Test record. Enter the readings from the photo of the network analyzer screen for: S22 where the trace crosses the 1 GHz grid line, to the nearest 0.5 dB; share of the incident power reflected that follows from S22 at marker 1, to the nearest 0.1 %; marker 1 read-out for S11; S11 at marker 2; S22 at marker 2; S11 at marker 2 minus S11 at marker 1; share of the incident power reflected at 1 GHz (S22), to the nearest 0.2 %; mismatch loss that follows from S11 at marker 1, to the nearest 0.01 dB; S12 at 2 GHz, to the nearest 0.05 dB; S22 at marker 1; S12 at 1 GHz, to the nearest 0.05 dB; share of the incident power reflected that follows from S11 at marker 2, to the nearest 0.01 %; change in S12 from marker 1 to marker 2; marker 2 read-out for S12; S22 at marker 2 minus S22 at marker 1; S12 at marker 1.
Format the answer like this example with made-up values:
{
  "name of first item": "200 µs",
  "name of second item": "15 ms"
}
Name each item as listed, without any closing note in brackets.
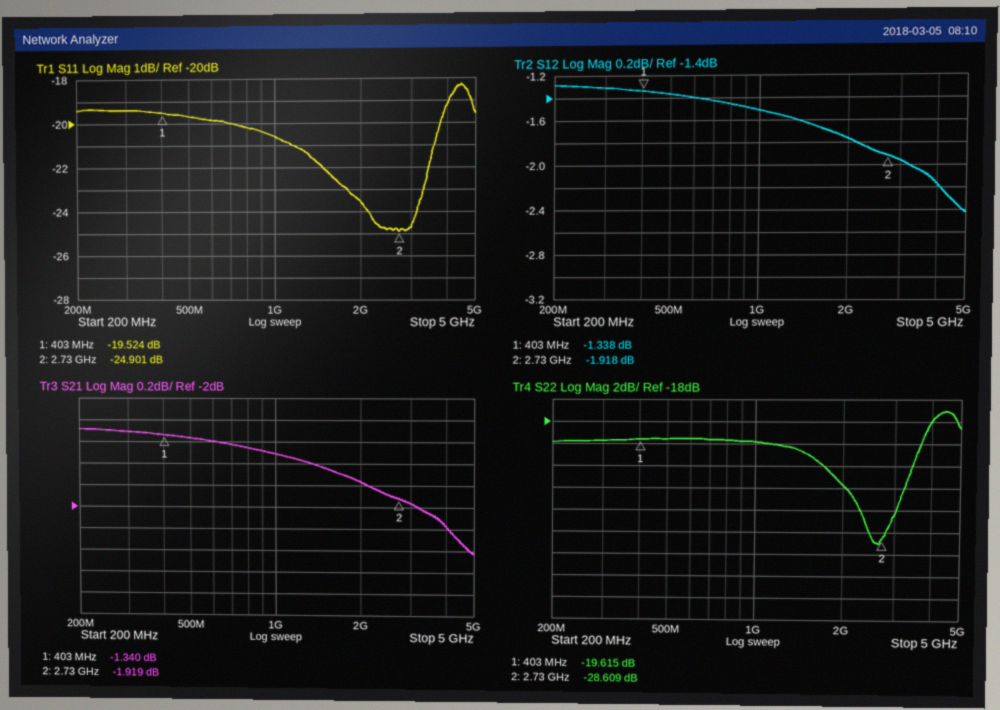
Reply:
{
  "S22 where the trace crosses the 1 GHz grid line, to the nearest 0.5 dB": "-20.0 dB",
  "share of the incident power reflected that follows from S22 at marker 1, to the nearest 0.1 %": "1.1 %",
  "marker 1 read-out for S11": "-19.524 dB",
  "S11 at marker 2": "-24.901 dB",
  "S22 at marker 2": "-28.609 dB",
  "S11 at marker 2 minus S11 at marker 1": "-5.377 dB",
  "share of the incident power reflected at 1 GHz (S22), to the nearest 0.2 %": "1.0 %",
  "mismatch loss that follows from S11 at marker 1, to the nearest 0.01 dB": "0.05 dB",
  "S12 at 2 GHz, to the nearest 0.05 dB": "-1.75 dB",
  "S22 at marker 1": "-19.615 dB",
  "S12 at 1 GHz, to the nearest 0.05 dB": "-1.50 dB",
  "share of the incident power reflected that follows from S11 at marker 2, to the nearest 0.01 %": "0.32 %",
  "change in S12 from marker 1 to marker 2": "-0.580 dB",
  "marker 2 read-out for S12": "-1.918 dB",
  "S22 at marker 2 minus S22 at marker 1": "-8.994 dB",
  "S12 at marker 1": "-1.338 dB"
}
